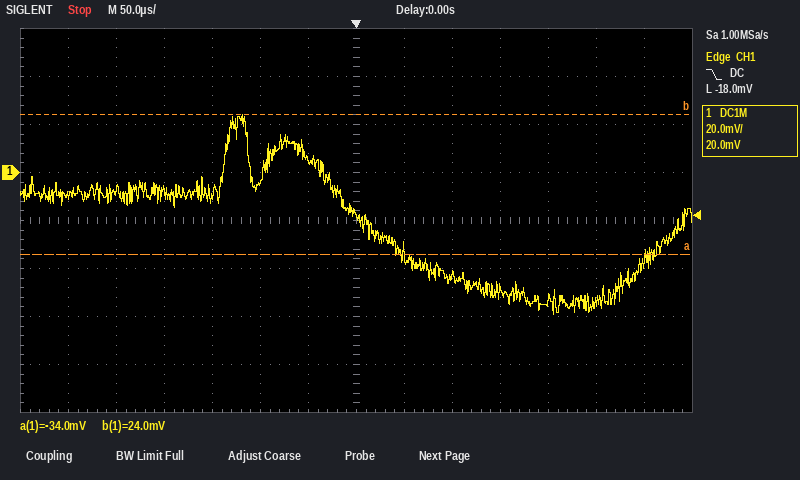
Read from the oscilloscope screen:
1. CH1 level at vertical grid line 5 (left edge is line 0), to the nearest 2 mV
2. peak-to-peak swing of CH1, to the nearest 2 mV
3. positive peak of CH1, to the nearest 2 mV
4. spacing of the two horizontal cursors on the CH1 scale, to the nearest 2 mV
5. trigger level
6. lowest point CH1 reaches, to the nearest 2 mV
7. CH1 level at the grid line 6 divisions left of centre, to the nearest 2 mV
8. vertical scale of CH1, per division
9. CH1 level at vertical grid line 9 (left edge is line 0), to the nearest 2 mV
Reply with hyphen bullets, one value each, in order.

- -4 mV
- 84 mV
- 24 mV
- 58 mV
- -18.0 mV
- -60 mV
- -10 mV
- 20 mV
- -42 mV
